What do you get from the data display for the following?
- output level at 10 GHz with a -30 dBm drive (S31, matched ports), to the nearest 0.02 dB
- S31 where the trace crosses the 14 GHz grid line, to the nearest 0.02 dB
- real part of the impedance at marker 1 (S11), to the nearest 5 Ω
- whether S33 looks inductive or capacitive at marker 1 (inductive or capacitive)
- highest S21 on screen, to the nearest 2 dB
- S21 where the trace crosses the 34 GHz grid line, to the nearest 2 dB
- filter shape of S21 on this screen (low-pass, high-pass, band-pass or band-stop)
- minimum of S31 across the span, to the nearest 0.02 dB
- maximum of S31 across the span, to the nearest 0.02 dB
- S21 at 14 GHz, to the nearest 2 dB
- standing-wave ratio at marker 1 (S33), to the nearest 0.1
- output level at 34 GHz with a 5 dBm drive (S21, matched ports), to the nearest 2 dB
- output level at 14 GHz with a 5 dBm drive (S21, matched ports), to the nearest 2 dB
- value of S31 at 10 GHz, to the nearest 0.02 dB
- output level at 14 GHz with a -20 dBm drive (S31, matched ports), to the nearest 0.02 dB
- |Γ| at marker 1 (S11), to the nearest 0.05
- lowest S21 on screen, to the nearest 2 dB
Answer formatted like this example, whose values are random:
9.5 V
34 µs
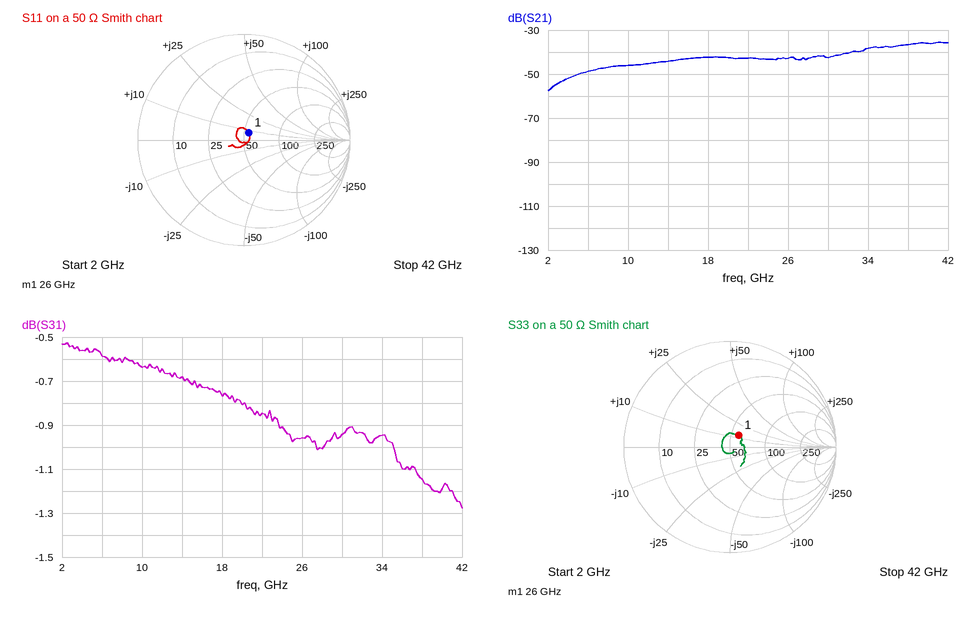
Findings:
-30.64 dBm
-0.68 dB
55 Ω
inductive
-36 dB
-38 dB
high-pass
-1.28 dB
-0.52 dB
-44 dB
1.3
-34 dBm
-40 dBm
-0.64 dB
-20.68 dBm
0.10
-58 dB
